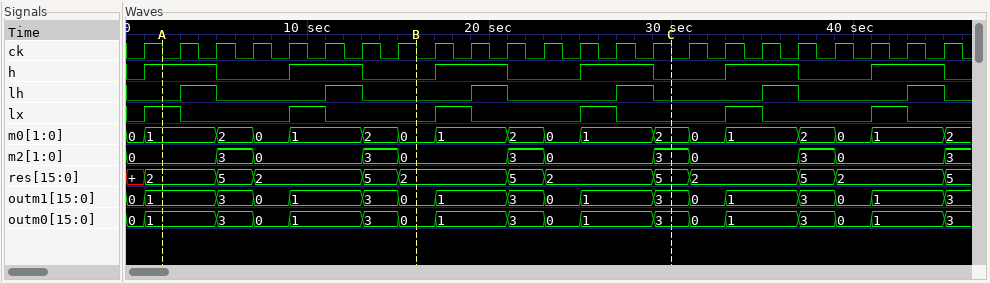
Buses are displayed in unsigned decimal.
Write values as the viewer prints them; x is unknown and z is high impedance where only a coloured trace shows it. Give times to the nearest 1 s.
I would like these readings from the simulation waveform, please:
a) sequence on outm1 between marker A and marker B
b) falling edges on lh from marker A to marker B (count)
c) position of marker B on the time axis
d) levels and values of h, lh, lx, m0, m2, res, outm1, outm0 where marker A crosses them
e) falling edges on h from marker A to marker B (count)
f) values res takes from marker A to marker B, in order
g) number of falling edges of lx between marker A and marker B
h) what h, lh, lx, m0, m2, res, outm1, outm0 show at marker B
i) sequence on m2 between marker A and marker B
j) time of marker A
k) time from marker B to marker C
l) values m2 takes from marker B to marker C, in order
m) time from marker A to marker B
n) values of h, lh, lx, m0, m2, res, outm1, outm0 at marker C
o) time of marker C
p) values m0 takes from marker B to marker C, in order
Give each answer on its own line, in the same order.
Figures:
1, 3, 0, 1, 3, 0
2
16 s
h=1, lh=0, lx=1, m0=1, m2=0, res=2, outm1=1, outm0=1
2
2, 5, 2, 5, 2
2
h=0, lh=0, lx=0, m0=0, m2=0, res=2, outm1=0, outm0=0
0, 3, 0, 3, 0
2 s
14 s
0, 3, 0, 3
14 s
h=0, lh=0, lx=0, m0=2, m2=3, res=5, outm1=3, outm0=3
30 s
0, 1, 2, 0, 1, 2
